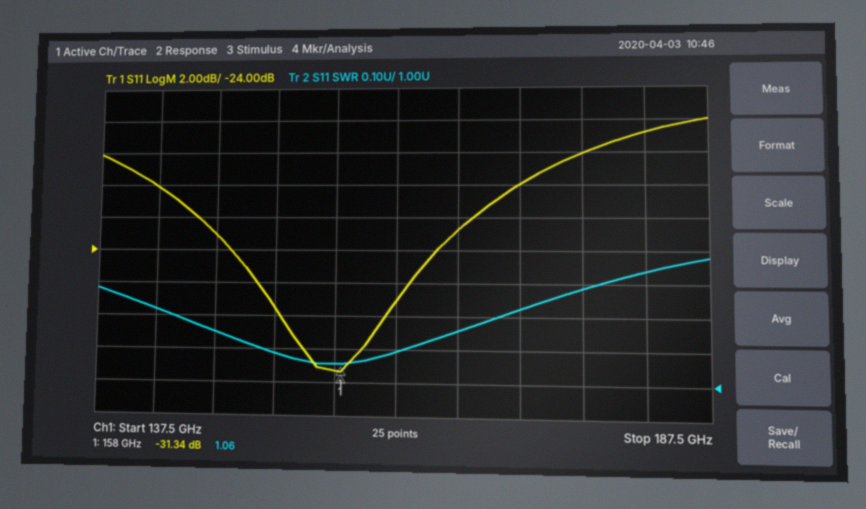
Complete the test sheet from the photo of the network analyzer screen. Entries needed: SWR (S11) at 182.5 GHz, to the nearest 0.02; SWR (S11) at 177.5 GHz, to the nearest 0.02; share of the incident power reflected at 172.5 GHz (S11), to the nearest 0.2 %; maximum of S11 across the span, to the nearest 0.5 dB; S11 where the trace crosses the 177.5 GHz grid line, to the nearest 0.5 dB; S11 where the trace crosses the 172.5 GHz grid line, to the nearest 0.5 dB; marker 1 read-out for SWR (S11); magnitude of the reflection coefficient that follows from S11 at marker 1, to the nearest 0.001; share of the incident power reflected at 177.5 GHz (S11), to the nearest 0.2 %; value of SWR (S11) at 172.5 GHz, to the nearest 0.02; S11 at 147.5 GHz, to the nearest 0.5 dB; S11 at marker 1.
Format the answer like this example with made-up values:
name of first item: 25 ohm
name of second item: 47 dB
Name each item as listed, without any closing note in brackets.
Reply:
SWR (S11) at 182.5 GHz, to the nearest 0.02: 1.34
SWR (S11) at 177.5 GHz, to the nearest 0.02: 1.28
share of the incident power reflected at 172.5 GHz (S11), to the nearest 0.2 %: 1.0 %
maximum of S11 across the span, to the nearest 0.5 dB: -16.0 dB
S11 where the trace crosses the 177.5 GHz grid line, to the nearest 0.5 dB: -18.0 dB
S11 where the trace crosses the 172.5 GHz grid line, to the nearest 0.5 dB: -20.0 dB
marker 1 read-out for SWR: 1.06
magnitude of the reflection coefficient that follows from S11 at marker 1, to the nearest 0.001: 0.027
share of the incident power reflected at 177.5 GHz (S11), to the nearest 0.2 %: 1.6 %
value of SWR (S11) at 172.5 GHz, to the nearest 0.02: 1.22
S11 at 147.5 GHz, to the nearest 0.5 dB: -23.0 dB
S11 at marker 1: -31.34 dB
